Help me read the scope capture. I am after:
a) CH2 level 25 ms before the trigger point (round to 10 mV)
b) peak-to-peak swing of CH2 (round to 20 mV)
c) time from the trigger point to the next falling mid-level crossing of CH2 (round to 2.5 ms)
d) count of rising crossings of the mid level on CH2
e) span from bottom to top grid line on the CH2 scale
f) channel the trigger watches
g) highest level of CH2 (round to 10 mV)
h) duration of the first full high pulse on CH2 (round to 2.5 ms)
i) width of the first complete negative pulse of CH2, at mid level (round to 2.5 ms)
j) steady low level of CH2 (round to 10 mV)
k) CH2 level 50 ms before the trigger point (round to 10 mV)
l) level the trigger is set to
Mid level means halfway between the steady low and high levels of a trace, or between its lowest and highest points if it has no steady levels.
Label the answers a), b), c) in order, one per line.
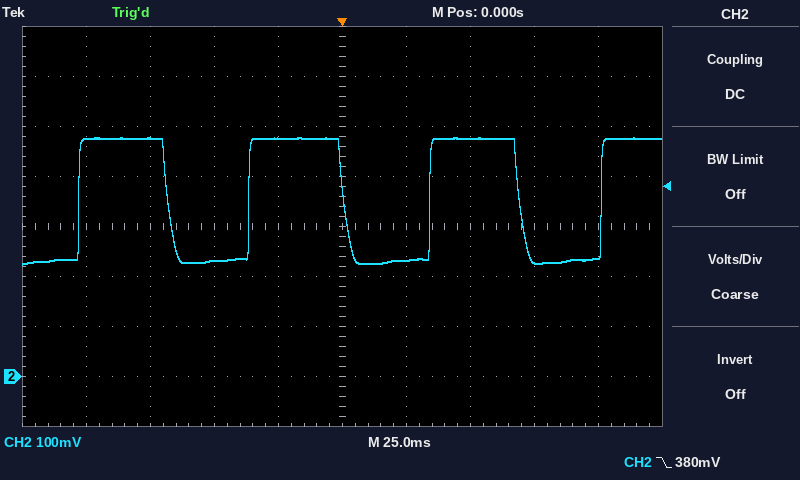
a) 480 mV
b) 260 mV
c) 70.0 ms
d) 4
e) 800 mV
f) CH2
g) 480 mV
h) 35.0 ms
i) 32.5 ms
j) 230 mV
k) 230 mV
l) 380 mV
